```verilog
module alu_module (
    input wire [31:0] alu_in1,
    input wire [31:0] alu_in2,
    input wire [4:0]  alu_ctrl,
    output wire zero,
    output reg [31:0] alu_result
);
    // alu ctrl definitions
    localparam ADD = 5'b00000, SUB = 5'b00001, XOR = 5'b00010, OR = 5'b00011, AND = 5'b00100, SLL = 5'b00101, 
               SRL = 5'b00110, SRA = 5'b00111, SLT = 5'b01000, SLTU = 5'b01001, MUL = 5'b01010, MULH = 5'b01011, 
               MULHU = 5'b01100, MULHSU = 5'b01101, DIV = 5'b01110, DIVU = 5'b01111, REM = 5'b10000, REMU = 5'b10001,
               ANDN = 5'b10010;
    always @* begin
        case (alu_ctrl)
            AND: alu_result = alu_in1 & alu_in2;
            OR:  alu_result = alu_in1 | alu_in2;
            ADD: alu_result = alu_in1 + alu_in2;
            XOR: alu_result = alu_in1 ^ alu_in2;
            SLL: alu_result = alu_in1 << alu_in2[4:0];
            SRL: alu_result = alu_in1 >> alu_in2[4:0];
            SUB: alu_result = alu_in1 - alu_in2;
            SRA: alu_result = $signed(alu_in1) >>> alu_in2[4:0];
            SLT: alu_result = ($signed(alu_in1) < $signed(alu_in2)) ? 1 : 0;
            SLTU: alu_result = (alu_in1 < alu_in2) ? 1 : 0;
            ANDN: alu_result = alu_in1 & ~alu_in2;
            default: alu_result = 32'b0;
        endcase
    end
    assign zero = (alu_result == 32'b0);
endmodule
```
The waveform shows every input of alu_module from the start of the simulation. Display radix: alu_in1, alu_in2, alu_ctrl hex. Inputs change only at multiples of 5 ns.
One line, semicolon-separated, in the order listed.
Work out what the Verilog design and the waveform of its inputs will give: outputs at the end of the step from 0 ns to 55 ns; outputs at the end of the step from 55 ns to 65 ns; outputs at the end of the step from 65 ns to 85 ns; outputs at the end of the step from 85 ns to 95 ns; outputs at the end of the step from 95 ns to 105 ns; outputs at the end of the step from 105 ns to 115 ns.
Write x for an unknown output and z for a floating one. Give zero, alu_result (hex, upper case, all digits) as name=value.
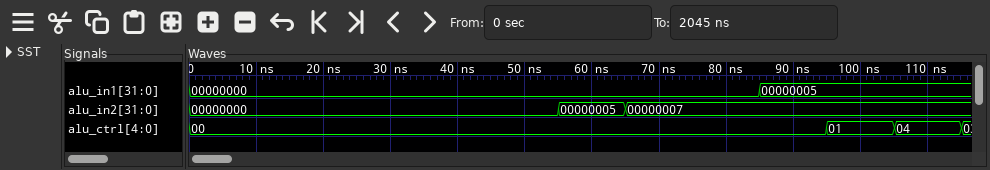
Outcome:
zero=1, alu_result=00000000; zero=0, alu_result=00000005; zero=0, alu_result=00000007; zero=0, alu_result=0000000C; zero=0, alu_result=FFFFFFFE; zero=0, alu_result=00000005
